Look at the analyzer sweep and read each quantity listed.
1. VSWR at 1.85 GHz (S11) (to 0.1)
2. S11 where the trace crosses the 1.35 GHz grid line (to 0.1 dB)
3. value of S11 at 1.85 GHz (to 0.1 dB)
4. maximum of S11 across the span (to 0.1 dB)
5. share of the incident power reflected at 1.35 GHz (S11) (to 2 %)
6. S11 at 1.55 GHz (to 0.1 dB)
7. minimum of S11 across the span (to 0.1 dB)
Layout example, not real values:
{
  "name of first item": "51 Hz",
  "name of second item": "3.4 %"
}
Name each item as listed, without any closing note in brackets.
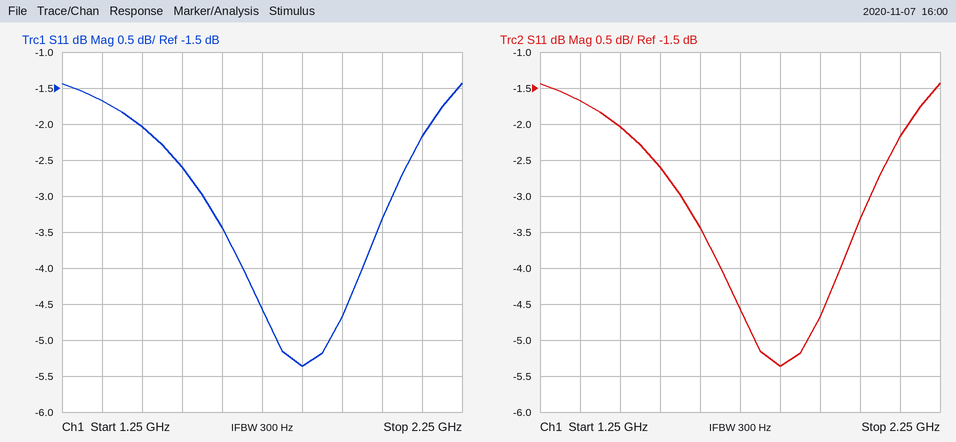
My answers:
{
  "VSWR at 1.85 GHz (S11)": "3.3",
  "S11 where the trace crosses the 1.35 GHz grid line": "-1.7 dB",
  "value of S11 at 1.85 GHz": "-5.4 dB",
  "maximum of S11 across the span": "-1.4 dB",
  "share of the incident power reflected at 1.35 GHz (S11)": "68 %",
  "S11 at 1.55 GHz": "-2.6 dB",
  "minimum of S11 across the span": "-5.4 dB"
}
